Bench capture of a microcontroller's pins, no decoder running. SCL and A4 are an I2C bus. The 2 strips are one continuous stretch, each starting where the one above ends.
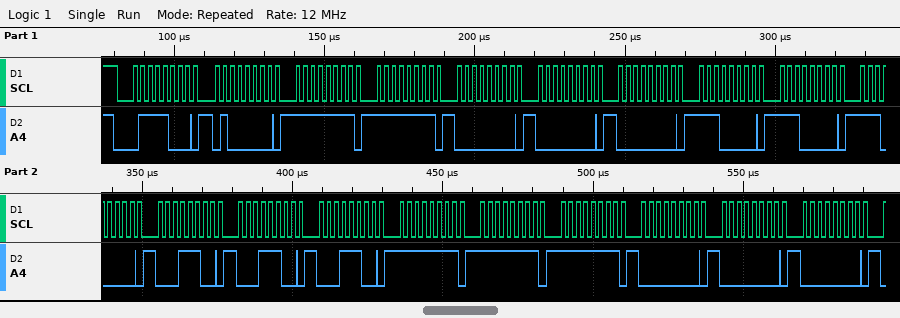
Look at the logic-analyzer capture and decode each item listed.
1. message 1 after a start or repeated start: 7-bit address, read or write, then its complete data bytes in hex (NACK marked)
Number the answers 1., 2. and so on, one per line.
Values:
1. 0x3C write: 40 FF FF 00 00 00 E0 E0 E0 1C 1C 1C FF FF FF 00 00 00
